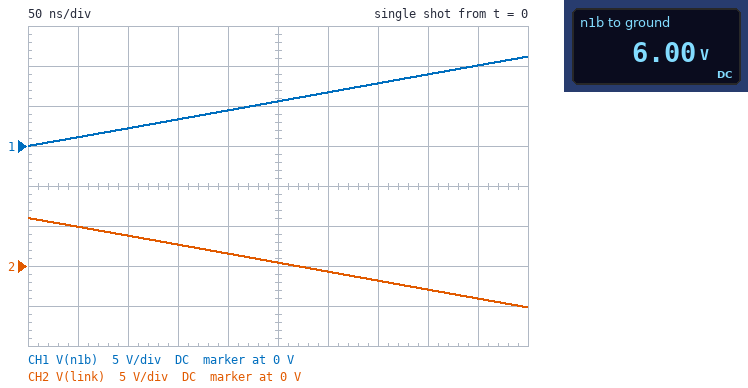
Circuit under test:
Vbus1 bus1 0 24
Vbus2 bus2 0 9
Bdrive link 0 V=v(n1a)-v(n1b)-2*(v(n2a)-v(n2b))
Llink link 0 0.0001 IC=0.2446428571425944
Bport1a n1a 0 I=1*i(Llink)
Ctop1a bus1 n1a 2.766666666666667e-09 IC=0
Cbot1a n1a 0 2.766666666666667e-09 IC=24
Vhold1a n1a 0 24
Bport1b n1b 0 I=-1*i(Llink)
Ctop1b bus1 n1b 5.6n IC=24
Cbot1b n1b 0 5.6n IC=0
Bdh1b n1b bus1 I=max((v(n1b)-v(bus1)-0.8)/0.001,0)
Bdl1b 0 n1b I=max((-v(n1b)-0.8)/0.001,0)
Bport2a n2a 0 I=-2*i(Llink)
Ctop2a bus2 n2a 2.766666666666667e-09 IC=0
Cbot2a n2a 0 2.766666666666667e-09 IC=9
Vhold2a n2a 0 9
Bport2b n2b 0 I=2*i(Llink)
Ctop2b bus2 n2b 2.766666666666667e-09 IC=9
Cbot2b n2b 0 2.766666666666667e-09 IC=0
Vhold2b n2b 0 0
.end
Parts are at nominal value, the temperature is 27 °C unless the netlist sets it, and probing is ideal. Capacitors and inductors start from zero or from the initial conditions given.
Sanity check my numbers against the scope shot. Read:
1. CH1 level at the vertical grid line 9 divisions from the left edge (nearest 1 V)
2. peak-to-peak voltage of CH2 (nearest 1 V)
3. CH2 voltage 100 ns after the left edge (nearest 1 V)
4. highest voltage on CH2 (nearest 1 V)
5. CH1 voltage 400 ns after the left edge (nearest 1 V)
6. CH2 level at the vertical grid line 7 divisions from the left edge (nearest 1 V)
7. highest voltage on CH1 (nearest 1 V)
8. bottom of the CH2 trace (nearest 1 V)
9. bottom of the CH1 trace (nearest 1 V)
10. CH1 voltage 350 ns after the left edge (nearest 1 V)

10 V
11 V
4 V
6 V
9 V
-2 V
11 V
-5 V
0 V
8 V
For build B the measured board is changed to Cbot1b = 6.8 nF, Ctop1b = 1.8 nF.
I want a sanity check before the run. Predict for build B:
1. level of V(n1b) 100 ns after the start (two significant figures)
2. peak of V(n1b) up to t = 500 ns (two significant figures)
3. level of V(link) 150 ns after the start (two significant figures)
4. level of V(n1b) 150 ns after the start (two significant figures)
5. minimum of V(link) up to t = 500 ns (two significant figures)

2.9 V
14 V
1.7 V
4.3 V
-8.4 V
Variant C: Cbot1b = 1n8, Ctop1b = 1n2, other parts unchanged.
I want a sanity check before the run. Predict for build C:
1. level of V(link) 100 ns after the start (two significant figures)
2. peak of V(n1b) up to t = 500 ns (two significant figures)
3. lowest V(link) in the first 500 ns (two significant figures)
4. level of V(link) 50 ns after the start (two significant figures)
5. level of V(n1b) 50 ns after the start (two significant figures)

-2.2 V
25 V
-19 V
1.9 V
4.1 V
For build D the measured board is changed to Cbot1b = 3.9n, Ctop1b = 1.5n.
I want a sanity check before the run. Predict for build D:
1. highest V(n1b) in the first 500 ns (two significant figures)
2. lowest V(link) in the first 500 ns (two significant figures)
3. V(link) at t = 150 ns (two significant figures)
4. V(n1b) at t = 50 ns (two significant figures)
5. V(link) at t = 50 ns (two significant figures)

22 V
-16 V
-870 mV
2.3 V
3.7 V
